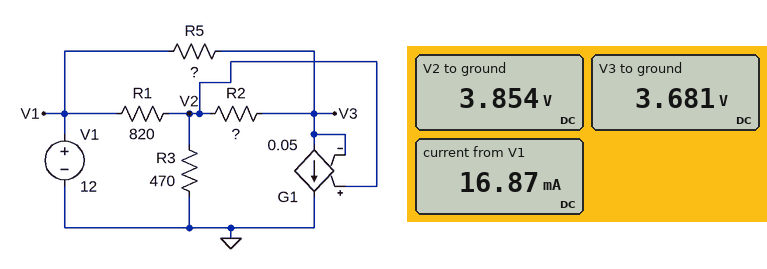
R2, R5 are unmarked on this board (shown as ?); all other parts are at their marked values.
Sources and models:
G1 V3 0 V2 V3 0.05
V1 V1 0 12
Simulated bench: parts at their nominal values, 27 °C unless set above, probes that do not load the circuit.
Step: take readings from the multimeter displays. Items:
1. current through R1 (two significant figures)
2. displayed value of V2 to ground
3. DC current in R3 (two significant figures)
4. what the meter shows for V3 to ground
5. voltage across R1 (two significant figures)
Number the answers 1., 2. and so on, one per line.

1. 9.9 mA
2. 3.854 V
3. 8.2 mA
4. 3.681 V
5. 8.1 V
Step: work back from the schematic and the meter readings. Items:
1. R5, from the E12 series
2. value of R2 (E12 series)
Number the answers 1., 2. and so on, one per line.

1. 1.2 kΩ
2. 100 Ω
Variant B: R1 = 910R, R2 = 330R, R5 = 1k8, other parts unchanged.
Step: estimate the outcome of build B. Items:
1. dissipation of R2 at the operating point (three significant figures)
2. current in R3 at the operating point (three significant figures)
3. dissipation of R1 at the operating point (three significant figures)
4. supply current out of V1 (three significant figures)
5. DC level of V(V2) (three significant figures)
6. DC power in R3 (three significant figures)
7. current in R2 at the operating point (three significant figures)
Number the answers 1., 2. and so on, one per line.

1. 27.8 µW
2. 8.50 mA
3. 70.4 mW
4. 13.3 mA
5. 4.00 V
6. 34.0 mW
7. 290 µA
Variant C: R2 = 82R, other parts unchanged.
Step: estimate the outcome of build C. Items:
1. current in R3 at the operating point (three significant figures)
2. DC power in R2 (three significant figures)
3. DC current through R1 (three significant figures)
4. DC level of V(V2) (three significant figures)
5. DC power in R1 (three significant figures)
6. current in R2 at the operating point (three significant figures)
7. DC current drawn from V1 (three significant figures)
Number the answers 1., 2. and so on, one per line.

1. 7.85 mA
2. 428 µW
3. 10.1 mA
4. 3.69 V
5. 84.2 mW
6. 2.28 mA
7. 17.2 mA
